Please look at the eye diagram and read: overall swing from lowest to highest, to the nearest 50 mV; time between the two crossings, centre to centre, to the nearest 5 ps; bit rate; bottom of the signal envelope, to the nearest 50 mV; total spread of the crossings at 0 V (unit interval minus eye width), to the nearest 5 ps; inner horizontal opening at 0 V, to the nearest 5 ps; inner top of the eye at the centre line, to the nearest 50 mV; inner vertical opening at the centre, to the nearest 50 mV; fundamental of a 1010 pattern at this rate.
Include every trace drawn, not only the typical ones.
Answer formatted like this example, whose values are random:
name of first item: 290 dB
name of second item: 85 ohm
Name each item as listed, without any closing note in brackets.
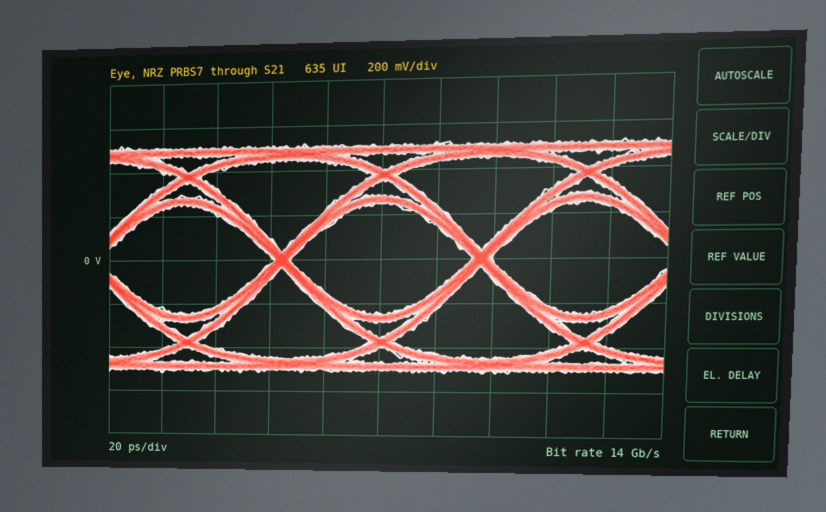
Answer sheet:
overall swing from lowest to highest, to the nearest 50 mV: 1.05 V
time between the two crossings, centre to centre, to the nearest 5 ps: 70 ps
bit rate: 14 Gb/s
bottom of the signal envelope, to the nearest 50 mV: -500 mV
total spread of the crossings at 0 V (unit interval minus eye width), to the nearest 5 ps: 5 ps
inner horizontal opening at 0 V, to the nearest 5 ps: 65 ps
inner top of the eye at the centre line, to the nearest 50 mV: 250 mV
inner vertical opening at the centre, to the nearest 50 mV: 500 mV
fundamental of a 1010 pattern at this rate: 7 GHz
